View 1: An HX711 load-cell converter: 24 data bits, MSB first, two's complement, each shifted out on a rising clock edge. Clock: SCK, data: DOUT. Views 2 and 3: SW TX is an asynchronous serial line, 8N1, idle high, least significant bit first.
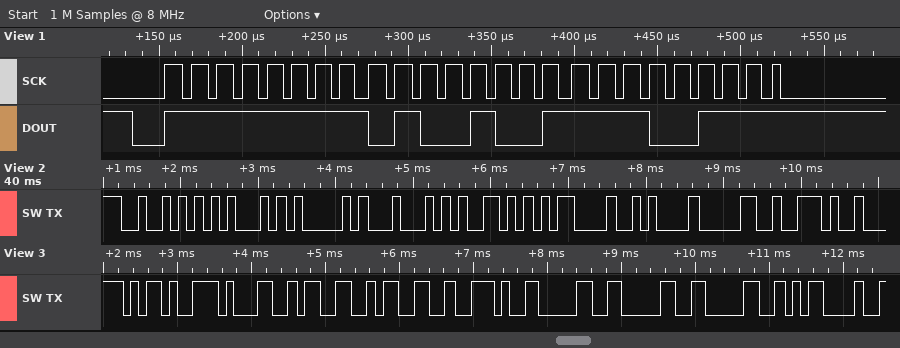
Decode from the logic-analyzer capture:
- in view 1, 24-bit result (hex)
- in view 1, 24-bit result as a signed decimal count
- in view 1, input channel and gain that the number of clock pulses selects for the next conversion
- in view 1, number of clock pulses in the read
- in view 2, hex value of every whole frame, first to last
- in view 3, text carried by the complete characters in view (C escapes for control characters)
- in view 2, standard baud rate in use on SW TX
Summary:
0xFF49E7
-46617
channel A, gain 128
25
52 45 41 44 59 0D 0A 30 2E
"-133.000\r"
9600 baud
